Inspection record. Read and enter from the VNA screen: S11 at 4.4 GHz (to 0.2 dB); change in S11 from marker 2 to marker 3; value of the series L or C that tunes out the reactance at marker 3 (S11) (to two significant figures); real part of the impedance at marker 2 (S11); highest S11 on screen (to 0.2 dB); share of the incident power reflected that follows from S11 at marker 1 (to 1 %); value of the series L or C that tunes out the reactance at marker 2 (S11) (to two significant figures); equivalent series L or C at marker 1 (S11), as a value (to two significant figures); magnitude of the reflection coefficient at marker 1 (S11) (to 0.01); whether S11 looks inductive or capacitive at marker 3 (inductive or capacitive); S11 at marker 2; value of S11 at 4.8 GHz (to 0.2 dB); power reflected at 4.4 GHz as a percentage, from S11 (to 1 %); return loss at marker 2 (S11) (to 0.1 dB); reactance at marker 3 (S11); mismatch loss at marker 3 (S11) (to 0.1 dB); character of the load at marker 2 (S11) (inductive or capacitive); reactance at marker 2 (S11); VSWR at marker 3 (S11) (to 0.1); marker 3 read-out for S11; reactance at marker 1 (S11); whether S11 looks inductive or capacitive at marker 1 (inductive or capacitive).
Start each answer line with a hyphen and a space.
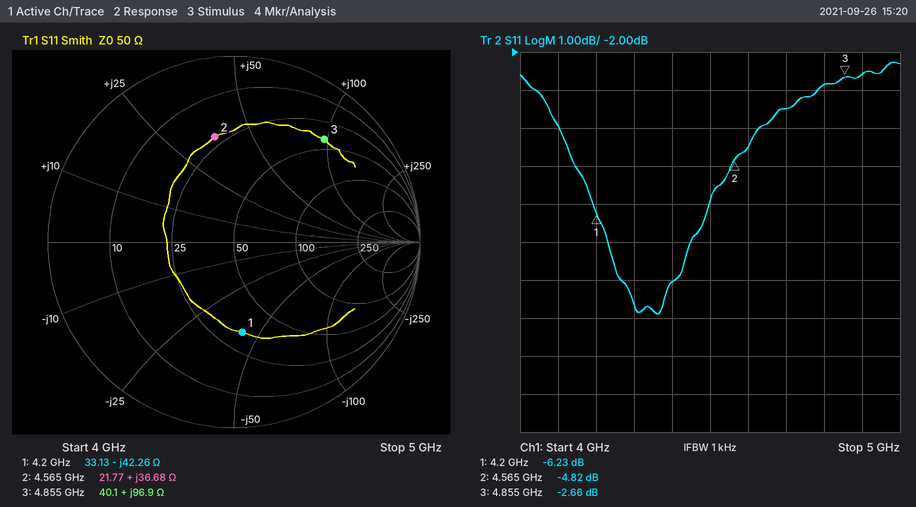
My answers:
- -8.0 dB
- 2.16 dB
- 340 fF
- 21.77 Ω
- -2.2 dB
- 24 %
- 950 fF
- 900 fF
- 0.49
- inductive
- -4.82 dB
- -2.8 dB
- 16 %
- 4.8 dB
- +96.9 Ω
- 3.4 dB
- inductive
- +36.68 Ω
- 6.6
- -2.66 dB
- -42.26 Ω
- capacitive
